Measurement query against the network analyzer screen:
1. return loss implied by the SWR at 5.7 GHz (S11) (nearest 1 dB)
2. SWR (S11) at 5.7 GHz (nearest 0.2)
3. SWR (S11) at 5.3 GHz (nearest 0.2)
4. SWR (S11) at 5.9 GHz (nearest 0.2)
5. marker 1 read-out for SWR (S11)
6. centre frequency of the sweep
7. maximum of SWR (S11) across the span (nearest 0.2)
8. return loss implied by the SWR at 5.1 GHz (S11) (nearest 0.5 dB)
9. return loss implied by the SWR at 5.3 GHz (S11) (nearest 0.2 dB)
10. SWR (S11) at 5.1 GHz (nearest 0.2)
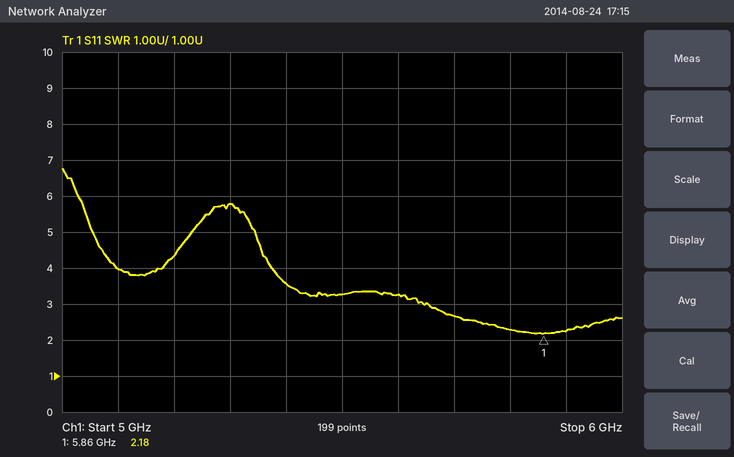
7 dB
2.6
5.8
2.2
2.18
5.5 GHz
6.8
4.5 dB
3.0 dB
4.0
